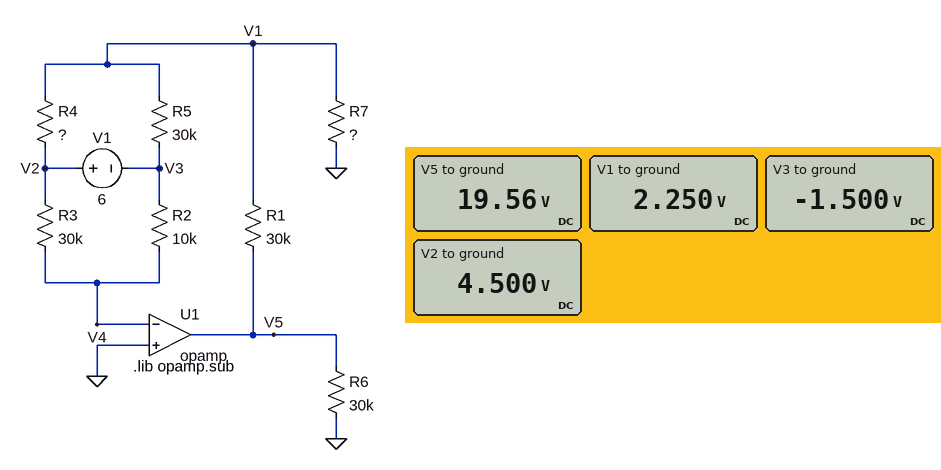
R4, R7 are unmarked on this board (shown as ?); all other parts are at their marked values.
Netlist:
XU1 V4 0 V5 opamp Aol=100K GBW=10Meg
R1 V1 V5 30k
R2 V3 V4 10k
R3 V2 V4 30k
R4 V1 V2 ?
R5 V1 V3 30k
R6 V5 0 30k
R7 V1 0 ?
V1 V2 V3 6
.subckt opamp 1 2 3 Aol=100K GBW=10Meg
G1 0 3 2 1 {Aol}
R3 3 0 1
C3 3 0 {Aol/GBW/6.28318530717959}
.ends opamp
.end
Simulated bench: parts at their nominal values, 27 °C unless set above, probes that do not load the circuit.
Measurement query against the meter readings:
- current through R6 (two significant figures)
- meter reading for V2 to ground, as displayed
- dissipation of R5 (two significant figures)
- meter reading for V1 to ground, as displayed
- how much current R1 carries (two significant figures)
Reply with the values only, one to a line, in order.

650 µA
4.500 V
470 µW
2.250 V
580 µA
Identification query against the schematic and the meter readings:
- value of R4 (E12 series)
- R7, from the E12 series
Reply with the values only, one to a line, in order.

18 kΩ
3.9 kΩ
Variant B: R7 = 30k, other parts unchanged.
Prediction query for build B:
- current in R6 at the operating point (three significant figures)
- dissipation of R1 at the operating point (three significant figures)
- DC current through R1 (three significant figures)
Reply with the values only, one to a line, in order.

150 µA
169 µW
75.0 µA
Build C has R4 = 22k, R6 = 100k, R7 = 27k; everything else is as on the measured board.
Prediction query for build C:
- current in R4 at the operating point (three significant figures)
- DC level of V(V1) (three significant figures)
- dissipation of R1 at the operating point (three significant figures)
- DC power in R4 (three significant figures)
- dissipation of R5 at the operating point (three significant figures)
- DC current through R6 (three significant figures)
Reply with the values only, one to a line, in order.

115 µA
1.96 V
158 µW
293 µW
399 µW
41.4 µA
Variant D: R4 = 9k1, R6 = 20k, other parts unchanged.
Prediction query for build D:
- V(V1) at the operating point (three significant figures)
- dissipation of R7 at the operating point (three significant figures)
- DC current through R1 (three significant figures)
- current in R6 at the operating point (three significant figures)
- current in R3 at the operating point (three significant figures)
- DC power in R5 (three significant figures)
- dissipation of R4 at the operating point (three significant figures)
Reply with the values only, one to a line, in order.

3.10 V
2.47 mW
796 µA
1.35 mA
150 µA
706 µW
214 µW
